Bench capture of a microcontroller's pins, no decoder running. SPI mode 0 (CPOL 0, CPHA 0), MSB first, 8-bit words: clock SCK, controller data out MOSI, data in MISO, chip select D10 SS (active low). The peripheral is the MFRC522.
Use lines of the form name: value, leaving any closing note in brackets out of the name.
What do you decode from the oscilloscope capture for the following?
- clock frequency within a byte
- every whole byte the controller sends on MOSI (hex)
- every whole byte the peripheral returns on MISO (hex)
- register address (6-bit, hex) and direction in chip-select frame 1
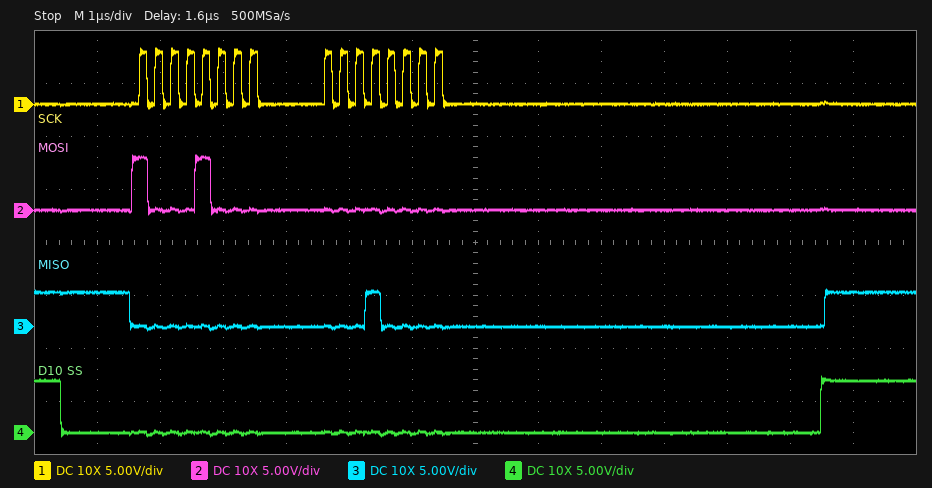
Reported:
clock frequency within a byte: 4 MHz
every whole byte the controller sends on MOSI: 88 00
every whole byte the peripheral returns on MISO: 00 10
register address (6-bit, hex) and direction in chip-select frame 1: 0x04 read
